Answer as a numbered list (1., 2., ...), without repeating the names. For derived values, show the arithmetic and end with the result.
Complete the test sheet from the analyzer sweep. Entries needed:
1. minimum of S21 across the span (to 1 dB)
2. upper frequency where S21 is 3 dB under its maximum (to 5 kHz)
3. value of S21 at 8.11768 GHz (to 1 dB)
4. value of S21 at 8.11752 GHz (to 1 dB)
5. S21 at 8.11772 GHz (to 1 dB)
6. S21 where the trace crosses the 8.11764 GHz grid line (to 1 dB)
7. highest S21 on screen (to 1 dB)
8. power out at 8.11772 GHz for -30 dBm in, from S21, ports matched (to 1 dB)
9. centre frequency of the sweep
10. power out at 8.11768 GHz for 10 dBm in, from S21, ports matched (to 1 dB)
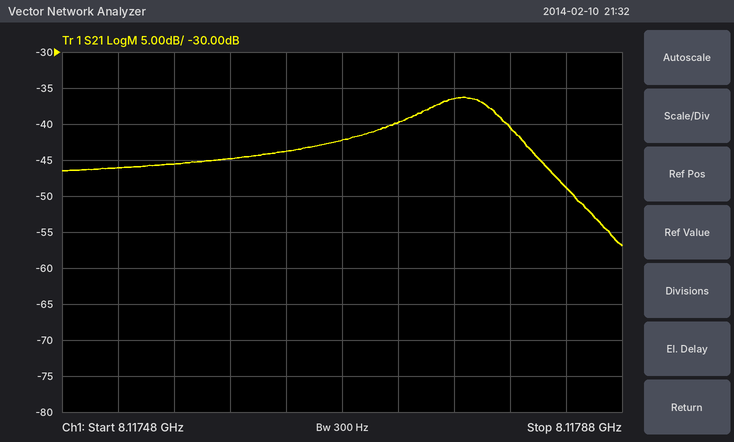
1. -57 dB
2. 8.117795 GHz
3. -42 dB
4. -46 dB
5. -40 dB
6. -44 dB
7. -36 dB
8. -30 dBm + (-40 dB) = -70 dBm
9. 8.11768 GHz
10. 10 dBm + (-42 dB) = -32 dBm
